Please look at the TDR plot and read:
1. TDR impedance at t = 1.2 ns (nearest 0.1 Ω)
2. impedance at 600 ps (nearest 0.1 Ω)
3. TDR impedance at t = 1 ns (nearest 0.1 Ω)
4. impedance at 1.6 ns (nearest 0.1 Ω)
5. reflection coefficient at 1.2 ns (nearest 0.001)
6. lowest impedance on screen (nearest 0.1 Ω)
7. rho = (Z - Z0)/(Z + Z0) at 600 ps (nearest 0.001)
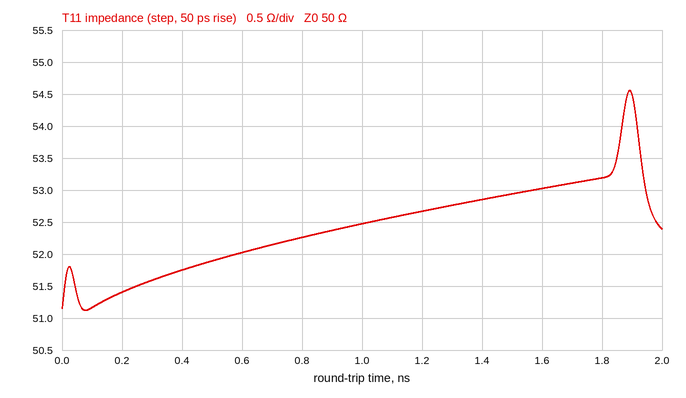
52.7 Ω
52.0 Ω
52.5 Ω
53.0 Ω
+0.026
51.1 Ω
+0.020
